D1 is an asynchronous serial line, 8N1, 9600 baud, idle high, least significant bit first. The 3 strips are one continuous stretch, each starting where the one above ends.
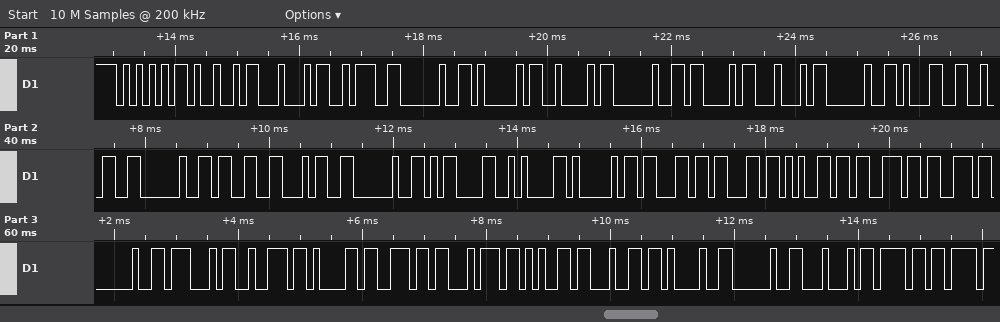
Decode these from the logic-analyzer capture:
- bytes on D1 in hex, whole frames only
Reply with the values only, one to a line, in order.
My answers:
55 49 44 3A 20 41 42 20 43 44 20 31 32 20 33 34 20 0D 0A 41 63 63 65 73 73 20 47 72 61 6E 74 65 64 21 20 44 6F
